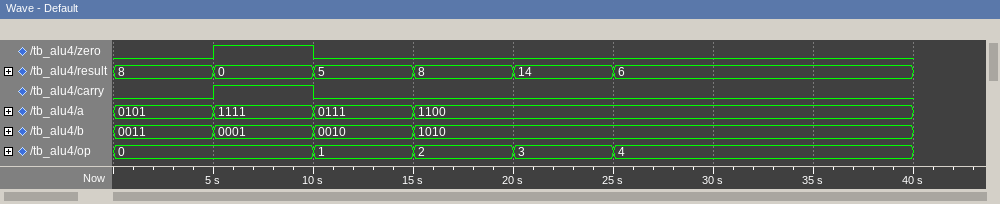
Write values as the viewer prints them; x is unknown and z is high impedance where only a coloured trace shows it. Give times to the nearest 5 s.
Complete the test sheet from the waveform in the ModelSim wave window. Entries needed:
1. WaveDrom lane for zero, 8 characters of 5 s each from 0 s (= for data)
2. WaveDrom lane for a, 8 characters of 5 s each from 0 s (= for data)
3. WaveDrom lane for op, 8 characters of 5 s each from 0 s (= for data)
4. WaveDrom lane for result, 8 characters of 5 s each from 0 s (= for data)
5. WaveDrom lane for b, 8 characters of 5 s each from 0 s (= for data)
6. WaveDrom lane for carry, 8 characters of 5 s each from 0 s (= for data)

{name: 'zero', wave: '010.....'}
{name: 'a', wave: '====....', data: '0101 1111 0111 1100'}
{name: 'op', wave: '=.====..', data: '0 1 2 3 4'}
{name: 'result', wave: '======..', data: '8 0 5 8 14 6'}
{name: 'b', wave: '====....', data: '0011 0001 0010 1010'}
{name: 'carry', wave: '010.....'}
